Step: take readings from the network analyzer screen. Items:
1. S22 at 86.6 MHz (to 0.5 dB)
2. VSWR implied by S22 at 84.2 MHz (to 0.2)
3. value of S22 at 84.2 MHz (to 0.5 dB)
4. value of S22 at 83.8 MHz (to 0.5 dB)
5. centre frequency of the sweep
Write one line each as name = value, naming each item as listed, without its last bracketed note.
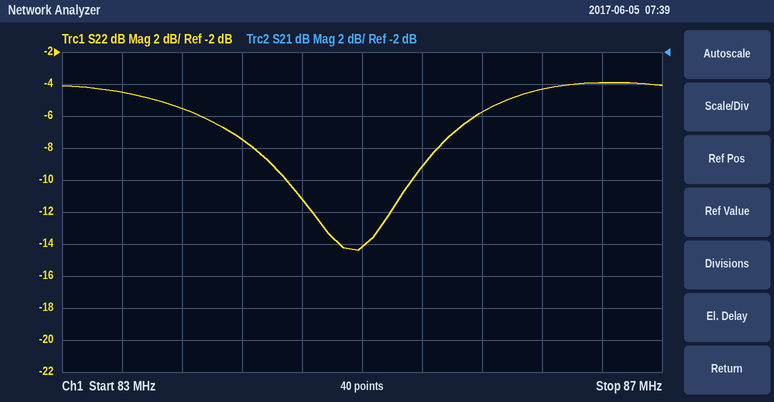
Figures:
S22 at 86.6 MHz = -4.0 dB
VSWR implied by S22 at 84.2 MHz = 2.4
value of S22 at 84.2 MHz = -7.5 dB
value of S22 at 83.8 MHz = -5.5 dB
centre frequency of the sweep = 85 MHz
